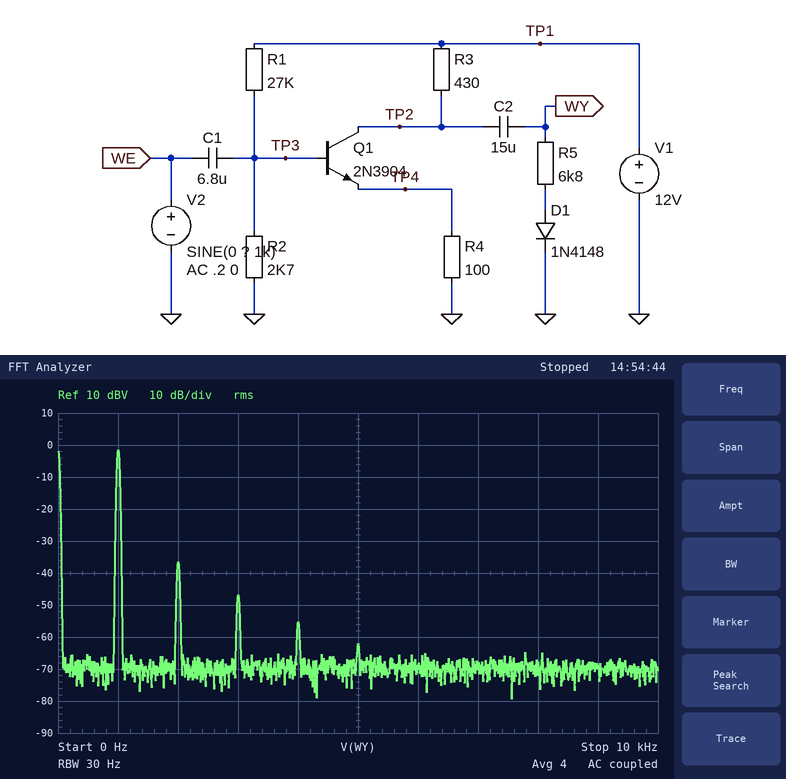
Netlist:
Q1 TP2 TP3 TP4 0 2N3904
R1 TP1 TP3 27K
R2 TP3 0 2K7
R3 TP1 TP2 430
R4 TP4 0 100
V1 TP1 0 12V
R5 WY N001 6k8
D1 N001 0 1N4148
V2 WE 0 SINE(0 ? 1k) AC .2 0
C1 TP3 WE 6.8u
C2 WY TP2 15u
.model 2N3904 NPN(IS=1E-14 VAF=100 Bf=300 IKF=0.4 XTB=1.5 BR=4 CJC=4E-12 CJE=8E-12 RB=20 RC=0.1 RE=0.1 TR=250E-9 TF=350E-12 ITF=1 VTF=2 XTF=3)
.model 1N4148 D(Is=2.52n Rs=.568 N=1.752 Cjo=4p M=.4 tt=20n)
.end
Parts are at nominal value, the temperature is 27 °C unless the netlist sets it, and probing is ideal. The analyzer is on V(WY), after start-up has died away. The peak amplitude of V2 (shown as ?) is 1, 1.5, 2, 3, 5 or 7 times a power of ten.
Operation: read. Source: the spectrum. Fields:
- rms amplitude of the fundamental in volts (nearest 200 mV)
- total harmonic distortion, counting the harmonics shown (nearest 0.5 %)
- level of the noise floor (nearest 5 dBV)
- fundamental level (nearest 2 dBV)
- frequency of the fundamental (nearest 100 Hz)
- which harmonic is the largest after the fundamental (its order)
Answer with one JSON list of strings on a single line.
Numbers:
["800 mV", "2.0 %", "-70 dBV", "-2 dBV", "1.0 kHz", "2"]
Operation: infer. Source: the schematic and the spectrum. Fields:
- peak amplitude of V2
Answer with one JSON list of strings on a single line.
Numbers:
["300 mV"]
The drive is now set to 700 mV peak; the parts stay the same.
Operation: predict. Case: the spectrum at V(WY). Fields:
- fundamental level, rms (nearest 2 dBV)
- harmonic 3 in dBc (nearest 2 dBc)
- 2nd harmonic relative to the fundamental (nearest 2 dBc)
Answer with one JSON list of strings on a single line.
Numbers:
["4 dBV", "-24 dBc", "-16 dBc"]
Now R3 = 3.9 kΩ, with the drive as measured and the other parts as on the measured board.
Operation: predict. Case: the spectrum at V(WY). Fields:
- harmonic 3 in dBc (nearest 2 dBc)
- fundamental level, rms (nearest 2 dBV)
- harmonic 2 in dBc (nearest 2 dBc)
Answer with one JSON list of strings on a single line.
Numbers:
["-16 dBc", "14 dBV", "-20 dBc"]
